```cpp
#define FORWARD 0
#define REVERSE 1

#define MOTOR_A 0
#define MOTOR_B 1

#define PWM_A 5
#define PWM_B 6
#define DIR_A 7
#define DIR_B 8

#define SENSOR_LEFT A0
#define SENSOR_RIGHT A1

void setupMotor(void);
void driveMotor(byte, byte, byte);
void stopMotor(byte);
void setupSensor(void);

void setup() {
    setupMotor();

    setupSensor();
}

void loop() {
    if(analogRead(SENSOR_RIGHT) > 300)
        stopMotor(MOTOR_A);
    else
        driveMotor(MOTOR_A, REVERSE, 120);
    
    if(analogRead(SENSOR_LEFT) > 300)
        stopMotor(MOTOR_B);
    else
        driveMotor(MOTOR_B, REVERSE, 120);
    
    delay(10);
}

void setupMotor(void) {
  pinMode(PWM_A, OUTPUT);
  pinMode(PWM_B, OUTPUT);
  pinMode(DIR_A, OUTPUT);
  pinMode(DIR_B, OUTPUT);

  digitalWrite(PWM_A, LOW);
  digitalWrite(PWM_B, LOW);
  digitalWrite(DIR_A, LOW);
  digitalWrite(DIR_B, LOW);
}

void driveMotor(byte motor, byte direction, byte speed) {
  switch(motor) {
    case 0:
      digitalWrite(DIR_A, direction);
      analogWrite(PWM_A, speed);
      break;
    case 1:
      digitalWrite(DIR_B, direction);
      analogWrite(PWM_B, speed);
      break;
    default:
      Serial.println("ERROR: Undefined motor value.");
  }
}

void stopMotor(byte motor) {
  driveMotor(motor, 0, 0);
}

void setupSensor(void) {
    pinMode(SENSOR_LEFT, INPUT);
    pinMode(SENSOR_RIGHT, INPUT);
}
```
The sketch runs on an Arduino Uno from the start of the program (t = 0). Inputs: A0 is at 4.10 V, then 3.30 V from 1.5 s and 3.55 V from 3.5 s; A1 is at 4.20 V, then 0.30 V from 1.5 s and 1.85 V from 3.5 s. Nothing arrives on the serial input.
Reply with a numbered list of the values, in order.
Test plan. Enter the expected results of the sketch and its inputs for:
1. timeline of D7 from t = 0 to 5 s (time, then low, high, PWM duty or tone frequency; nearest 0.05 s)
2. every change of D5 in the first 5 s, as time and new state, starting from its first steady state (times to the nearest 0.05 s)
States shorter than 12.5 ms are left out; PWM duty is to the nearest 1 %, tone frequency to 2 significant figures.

1. 0 s low; 1.5 s high; 3.5 s low
2. 0 s low; 1.5 s PWM 47 %; 3.5 s low
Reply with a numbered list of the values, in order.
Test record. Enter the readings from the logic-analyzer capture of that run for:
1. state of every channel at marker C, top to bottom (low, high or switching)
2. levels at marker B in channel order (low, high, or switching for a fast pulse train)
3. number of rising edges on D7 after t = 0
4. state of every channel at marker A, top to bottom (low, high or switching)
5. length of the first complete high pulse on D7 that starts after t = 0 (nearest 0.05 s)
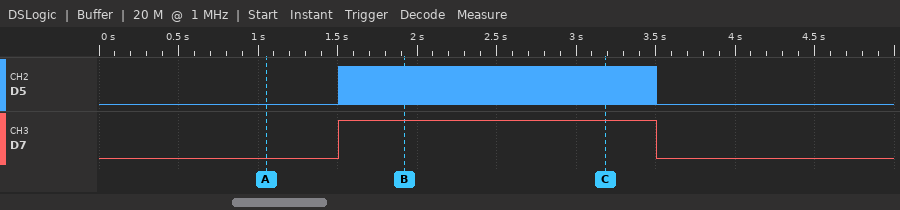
1. D5 switching, D7 high
2. D5 switching, D7 high
3. 1
4. D5 low, D7 low
5. 2.00 s
